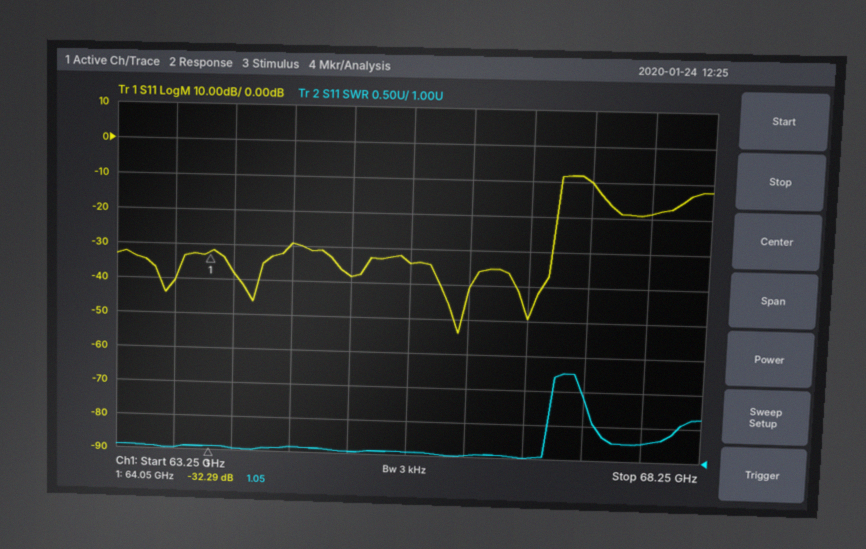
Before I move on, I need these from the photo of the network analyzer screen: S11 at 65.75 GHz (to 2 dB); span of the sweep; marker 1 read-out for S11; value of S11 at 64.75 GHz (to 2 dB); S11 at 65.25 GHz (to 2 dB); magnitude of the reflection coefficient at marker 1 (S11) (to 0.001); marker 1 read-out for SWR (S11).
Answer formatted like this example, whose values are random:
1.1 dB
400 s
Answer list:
-34 dB
5 GHz
-32.29 dB
-30 dB
-38 dB
0.024
1.05
